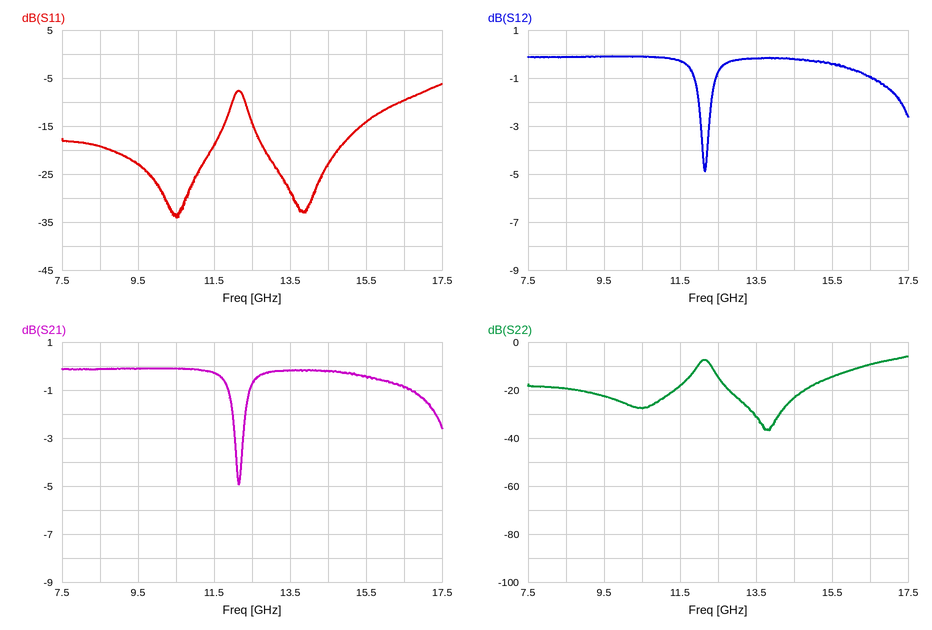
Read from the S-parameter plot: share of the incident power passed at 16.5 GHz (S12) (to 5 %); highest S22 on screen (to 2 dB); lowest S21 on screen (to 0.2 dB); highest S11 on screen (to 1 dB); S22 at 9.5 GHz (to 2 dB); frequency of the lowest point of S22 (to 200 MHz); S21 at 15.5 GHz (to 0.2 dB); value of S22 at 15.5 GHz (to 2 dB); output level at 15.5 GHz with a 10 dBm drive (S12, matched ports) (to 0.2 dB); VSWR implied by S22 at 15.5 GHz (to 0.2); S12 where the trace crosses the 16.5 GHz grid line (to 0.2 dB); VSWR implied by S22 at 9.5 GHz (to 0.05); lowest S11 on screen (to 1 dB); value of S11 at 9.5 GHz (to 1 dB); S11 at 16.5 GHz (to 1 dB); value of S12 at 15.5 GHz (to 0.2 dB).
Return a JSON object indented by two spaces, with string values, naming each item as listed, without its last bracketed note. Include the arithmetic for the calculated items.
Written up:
{
  "share of the incident power passed at 16.5 GHz (S12)": "10^(-1/10) ≈ 79.4 %, so 80 % to the nearest 5 %",
  "highest S22 on screen": "-6 dB",
  "lowest S21 on screen": "-5.0 dB",
  "highest S11 on screen": "-6 dB",
  "S22 at 9.5 GHz": "-22 dB",
  "frequency of the lowest point of S22": "13.8 GHz",
  "S21 at 15.5 GHz": "-0.4 dB",
  "value of S22 at 15.5 GHz": "-14 dB",
  "output level at 15.5 GHz with a 10 dBm drive (S12, matched ports)": "10 dBm + (-0.4 dB) = 9.6 dBm",
  "VSWR implied by S22 at 15.5 GHz": "|Γ| = 10^(-14/20) = 0.1995; VSWR = (1 + 0.1995)/(1 − 0.1995) ≈ 1.50, so 1.4 to the nearest 0.2",
  "S12 where the trace crosses the 16.5 GHz grid line": "-1.0 dB",
  "VSWR implied by S22 at 9.5 GHz": "|Γ| = 10^(-22/20) = 0.0794; VSWR = (1 + 0.0794)/(1 − 0.0794) ≈ 1.17, so 1.15 to the nearest 0.05",
  "lowest S11 on screen": "-34 dB",
  "value of S11 at 9.5 GHz": "-23 dB",
  "S11 at 16.5 GHz": "-10 dB",
  "value of S12 at 15.5 GHz": "-0.4 dB"
}
